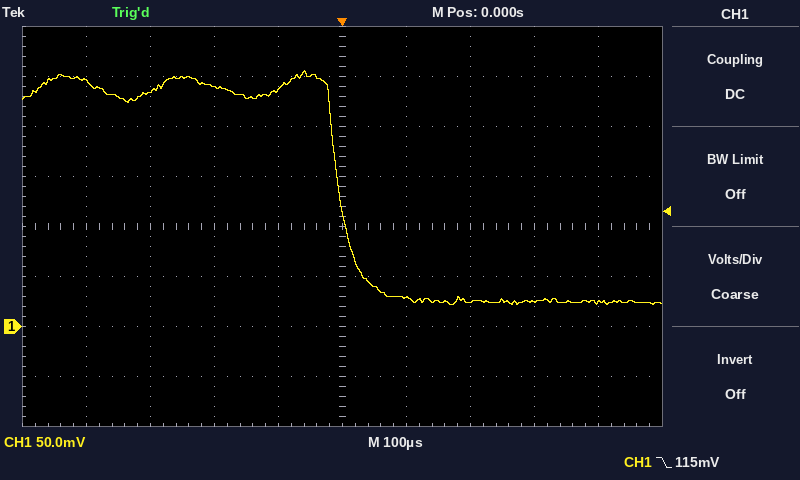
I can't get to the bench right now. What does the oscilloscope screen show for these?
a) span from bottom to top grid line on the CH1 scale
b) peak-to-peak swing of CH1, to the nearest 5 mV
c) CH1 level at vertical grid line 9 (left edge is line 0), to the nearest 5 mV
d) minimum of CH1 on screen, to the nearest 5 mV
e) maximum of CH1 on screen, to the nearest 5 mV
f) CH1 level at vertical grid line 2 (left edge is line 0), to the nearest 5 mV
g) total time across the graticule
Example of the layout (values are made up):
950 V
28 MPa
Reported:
400 mV
235 mV
25 mV
20 mV
255 mV
235 mV
1 ms
